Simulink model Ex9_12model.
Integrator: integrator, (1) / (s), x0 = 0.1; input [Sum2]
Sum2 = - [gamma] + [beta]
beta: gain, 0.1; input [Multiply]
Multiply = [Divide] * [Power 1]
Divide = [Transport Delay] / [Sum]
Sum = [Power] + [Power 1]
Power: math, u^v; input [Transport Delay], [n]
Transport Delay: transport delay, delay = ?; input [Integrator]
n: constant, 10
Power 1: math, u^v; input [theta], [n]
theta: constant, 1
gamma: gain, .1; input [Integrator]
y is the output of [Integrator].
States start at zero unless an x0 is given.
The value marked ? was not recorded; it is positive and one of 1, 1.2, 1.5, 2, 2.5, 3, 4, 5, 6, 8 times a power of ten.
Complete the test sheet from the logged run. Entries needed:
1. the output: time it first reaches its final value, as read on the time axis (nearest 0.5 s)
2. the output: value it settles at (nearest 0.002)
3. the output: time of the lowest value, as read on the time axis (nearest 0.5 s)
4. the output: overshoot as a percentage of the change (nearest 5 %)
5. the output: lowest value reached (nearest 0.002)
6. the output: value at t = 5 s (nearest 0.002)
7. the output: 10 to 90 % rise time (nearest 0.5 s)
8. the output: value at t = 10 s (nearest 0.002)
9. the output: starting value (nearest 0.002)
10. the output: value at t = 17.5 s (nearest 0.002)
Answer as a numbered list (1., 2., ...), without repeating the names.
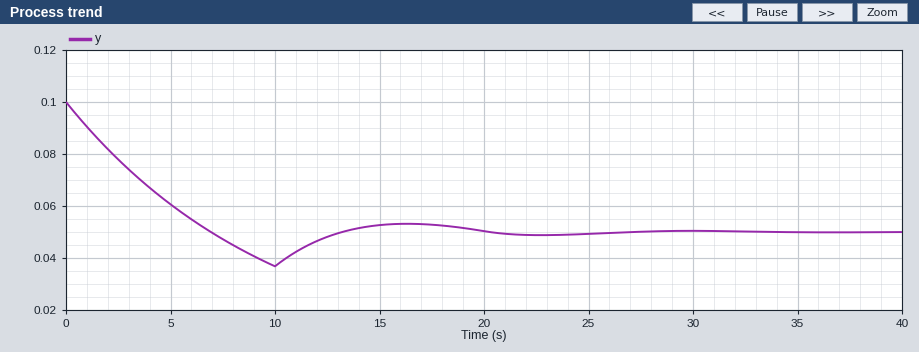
1. 7.0 s
2. 0.050
3. 10.0 s
4. 25 %
5. 0.036
6. 0.060
7. 5.5 s
8. 0.036
9. 0.100
10. 0.052
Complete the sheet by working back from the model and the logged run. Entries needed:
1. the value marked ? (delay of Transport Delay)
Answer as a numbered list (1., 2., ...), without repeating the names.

1. 10
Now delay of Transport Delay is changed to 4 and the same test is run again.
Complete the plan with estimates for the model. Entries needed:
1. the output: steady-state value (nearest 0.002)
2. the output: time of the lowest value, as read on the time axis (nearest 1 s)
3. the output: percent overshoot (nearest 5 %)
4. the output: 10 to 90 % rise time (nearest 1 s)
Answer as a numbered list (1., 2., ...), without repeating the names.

1. 0.072
2. 4 s
3. 15 %
4. 3 s
